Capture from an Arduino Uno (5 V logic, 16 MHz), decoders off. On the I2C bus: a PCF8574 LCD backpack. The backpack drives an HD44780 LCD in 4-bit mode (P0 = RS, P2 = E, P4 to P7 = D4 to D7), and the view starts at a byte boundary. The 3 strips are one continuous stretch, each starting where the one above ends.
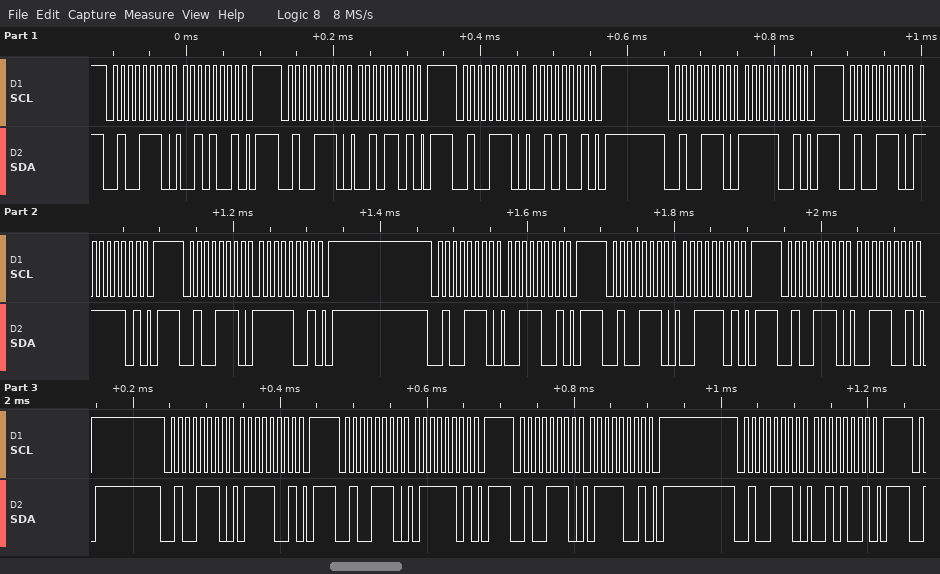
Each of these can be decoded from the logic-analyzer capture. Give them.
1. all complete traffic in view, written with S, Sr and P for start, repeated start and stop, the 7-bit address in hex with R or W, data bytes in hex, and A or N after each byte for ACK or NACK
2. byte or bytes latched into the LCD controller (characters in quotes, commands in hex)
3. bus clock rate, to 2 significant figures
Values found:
S 27W A 29 A P S 27W A 2D A P S 27W A 29 A P S 27W A F9 A P S 27W A FD A P S 27W A F9 A P S 27W A 39 A P S 27W A 3D A P S 27W A 39 A P S 27W A 79 A P S 27W A 7D A P S 27W A 79 A P S 27W A 29 A P
'/' '7'
100 kHz
